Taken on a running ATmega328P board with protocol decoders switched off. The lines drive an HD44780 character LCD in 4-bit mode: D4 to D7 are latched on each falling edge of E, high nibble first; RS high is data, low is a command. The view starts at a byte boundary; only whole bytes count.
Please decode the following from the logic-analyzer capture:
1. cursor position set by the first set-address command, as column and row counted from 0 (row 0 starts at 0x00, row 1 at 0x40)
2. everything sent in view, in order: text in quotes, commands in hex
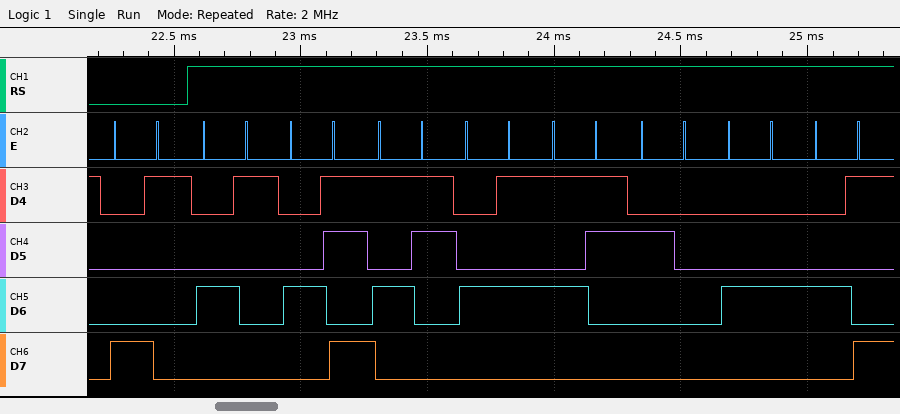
column 1, row 0
0x81 "AKSES DI"
